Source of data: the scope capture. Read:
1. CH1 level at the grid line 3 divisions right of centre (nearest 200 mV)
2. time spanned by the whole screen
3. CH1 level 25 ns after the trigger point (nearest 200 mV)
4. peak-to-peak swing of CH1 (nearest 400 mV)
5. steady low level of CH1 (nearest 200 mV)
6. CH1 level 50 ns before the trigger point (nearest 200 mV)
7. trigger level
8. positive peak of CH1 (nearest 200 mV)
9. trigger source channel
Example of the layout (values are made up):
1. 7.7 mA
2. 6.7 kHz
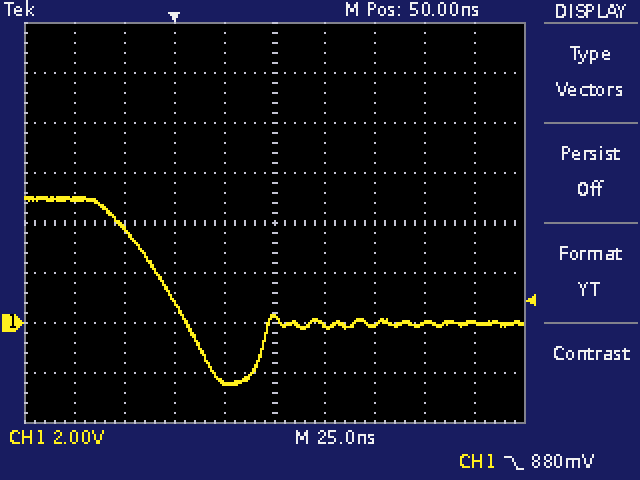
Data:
1. 0.0 V
2. 250 ns
3. -2.4 V
4. 7.6 V
5. 0.0 V
6. 5.0 V
7. 880 mV
8. 5.0 V
9. CH1
